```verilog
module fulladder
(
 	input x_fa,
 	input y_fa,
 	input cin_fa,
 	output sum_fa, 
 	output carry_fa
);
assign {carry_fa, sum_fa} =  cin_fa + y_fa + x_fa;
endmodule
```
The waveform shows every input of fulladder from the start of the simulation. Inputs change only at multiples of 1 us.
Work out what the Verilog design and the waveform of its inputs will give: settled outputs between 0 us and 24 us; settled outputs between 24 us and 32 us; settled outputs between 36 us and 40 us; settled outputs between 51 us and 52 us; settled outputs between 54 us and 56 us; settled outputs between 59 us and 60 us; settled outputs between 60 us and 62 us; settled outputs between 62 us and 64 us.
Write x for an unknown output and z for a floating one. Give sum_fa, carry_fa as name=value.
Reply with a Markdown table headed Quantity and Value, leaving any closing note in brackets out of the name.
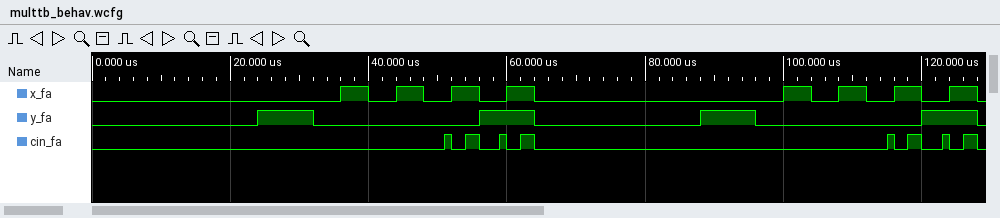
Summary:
| Quantity | Value |
|---|---|
| settled outputs between 0 us and 24 us | sum_fa=0, carry_fa=0 |
| settled outputs between 24 us and 32 us | sum_fa=1, carry_fa=0 |
| settled outputs between 36 us and 40 us | sum_fa=1, carry_fa=0 |
| settled outputs between 51 us and 52 us | sum_fa=1, carry_fa=0 |
| settled outputs between 54 us and 56 us | sum_fa=0, carry_fa=1 |
| settled outputs between 59 us and 60 us | sum_fa=0, carry_fa=1 |
| settled outputs between 60 us and 62 us | sum_fa=0, carry_fa=1 |
| settled outputs between 62 us and 64 us | sum_fa=1, carry_fa=1 |
